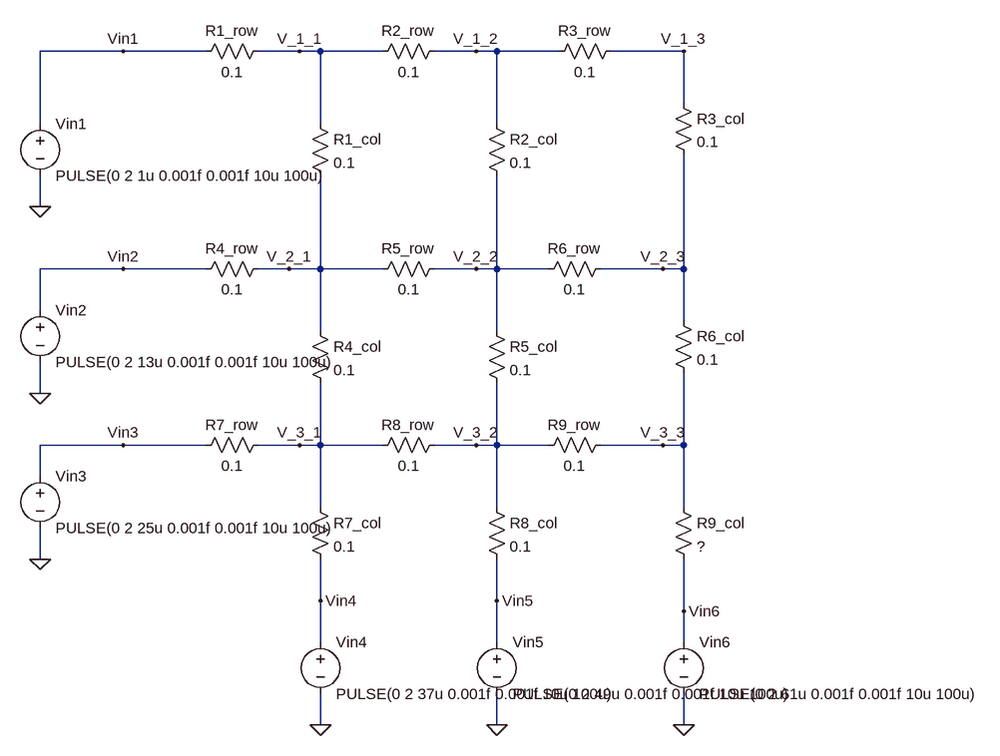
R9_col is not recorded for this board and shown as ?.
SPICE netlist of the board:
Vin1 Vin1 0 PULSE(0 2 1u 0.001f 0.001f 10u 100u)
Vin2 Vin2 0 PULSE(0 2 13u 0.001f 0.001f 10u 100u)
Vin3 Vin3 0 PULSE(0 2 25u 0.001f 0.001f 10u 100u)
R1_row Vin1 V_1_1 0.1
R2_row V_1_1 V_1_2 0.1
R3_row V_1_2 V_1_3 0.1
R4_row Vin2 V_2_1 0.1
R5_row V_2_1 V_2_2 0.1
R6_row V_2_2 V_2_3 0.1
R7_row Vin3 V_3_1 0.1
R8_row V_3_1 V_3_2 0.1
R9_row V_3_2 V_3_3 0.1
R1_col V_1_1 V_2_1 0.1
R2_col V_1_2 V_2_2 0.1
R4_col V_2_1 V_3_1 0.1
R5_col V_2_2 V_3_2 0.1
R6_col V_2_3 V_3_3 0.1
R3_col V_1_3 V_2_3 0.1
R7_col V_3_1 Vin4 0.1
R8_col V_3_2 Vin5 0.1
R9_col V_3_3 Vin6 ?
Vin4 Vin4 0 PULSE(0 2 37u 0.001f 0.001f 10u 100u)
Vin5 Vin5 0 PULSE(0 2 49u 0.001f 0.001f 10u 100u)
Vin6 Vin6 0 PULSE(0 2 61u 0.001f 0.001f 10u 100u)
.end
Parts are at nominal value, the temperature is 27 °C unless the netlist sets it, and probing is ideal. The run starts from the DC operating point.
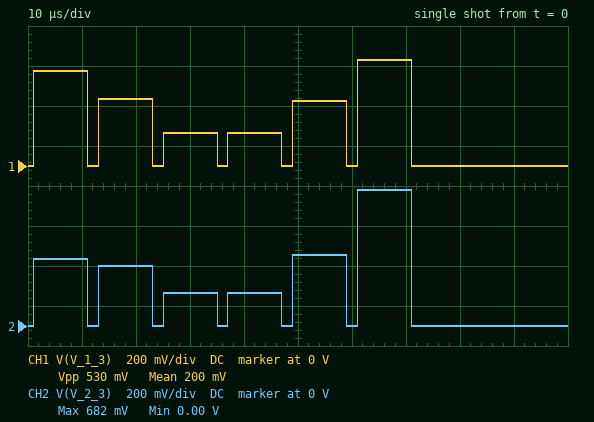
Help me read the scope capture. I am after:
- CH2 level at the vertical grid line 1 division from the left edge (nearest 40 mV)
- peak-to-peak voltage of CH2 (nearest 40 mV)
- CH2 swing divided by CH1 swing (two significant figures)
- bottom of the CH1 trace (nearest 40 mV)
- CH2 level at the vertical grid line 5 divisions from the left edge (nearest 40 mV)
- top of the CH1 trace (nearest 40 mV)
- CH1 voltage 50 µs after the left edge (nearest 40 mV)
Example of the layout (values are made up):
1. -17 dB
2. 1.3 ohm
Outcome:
1. 320 mV
2. 680 mV
3. 1.3
4. 0 V
5. 360 mV
6. 520 mV
7. 320 mV
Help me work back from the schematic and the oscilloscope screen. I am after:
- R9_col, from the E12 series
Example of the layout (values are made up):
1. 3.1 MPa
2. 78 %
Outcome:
1. 0.082 Ω
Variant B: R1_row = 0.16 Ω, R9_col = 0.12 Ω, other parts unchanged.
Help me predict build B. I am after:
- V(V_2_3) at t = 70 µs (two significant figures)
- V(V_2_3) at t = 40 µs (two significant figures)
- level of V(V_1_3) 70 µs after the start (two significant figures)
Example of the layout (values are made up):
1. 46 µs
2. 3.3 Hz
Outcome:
1. 580 mV
2. 190 mV
3. 460 mV
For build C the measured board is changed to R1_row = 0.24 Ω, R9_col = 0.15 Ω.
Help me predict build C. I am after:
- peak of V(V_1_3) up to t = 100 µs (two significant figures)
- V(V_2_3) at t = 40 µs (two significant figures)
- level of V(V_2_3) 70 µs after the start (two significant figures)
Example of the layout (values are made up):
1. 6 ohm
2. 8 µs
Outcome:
1. 440 mV
2. 210 mV
3. 520 mV
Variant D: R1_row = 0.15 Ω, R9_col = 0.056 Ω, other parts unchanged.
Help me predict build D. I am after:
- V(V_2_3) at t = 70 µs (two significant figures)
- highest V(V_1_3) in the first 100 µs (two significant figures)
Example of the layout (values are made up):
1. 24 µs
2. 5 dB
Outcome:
1. 810 mV
2. 640 mV
